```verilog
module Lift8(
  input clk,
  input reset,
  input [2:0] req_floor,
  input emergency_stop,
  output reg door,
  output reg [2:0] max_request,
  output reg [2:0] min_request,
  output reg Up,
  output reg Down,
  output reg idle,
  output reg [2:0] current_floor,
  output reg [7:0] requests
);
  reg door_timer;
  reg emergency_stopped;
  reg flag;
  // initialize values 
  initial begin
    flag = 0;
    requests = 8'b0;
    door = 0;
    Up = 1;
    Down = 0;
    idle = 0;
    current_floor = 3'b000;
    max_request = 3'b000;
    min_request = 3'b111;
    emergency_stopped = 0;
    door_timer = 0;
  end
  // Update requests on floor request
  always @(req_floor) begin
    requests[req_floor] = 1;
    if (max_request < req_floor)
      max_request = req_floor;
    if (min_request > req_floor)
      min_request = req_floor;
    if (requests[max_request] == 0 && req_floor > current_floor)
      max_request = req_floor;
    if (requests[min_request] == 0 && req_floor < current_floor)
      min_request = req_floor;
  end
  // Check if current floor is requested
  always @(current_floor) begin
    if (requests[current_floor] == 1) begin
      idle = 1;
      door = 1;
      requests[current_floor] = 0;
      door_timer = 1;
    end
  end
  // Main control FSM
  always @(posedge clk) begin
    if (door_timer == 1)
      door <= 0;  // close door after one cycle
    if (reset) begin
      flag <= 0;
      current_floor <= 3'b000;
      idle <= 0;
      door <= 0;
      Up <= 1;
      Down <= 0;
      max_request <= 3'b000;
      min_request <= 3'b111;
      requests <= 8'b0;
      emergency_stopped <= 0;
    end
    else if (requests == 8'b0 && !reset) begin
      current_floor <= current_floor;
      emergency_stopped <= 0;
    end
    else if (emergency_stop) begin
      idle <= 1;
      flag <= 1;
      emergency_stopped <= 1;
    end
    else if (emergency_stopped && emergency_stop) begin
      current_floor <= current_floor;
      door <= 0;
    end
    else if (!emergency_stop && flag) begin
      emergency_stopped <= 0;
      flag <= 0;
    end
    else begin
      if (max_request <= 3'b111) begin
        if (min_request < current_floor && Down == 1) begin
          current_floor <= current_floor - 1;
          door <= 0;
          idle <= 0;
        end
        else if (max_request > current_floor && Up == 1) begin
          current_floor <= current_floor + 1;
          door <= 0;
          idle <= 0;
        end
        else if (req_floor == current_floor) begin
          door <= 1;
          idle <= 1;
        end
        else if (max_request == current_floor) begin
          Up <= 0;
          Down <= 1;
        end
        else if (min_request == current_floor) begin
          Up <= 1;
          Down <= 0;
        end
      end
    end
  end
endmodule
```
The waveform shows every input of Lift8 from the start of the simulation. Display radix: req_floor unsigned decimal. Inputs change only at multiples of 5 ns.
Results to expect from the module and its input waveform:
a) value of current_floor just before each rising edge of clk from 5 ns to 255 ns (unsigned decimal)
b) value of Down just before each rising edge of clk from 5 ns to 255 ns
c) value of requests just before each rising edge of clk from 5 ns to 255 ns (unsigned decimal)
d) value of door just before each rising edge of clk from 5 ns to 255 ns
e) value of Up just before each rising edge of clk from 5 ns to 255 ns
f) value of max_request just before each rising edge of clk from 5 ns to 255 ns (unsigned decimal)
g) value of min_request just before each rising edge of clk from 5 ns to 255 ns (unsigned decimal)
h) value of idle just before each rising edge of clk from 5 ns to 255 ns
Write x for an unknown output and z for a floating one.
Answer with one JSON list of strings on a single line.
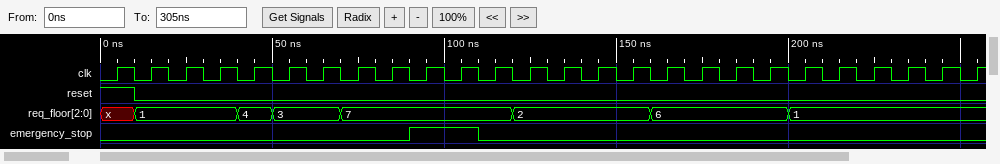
["0, 0, 1, 1, 1, 2, 3, 4, 5, 6, 6, 6, 6, 7, 7, 6, 5, 4, 3, 2, 2, 3, 4, 5, 6, 6", "0 0 0 0 0 0 0 0 0 0 0 0 0 0 1 1 1 1 1 1 0 0 0 0 0 1", "0, 2, 0, 0, 16, 24, 16, 128, 128, 128, 128, 128, 132, 4, 4, 4, 68, 68, 68, 64, 66, 66, 66, 66, 2, 2", "0 0 1 0 0 0 1 1 0 0 0 0 0 1 0 0 0 0 0 1 0 0 0 0 1 0", "1 1 1 1 1 1 1 1 1 1 1 1 1 1 0 0 0 0 0 0 1 1 1 1 1 0", "0, 1, 1, 1, 4, 4, 4, 7, 7, 7, 7, 7, 7, 7, 7, 7, 6, 6, 6, 6, 6, 6, 6, 6, 6, 6", "7, 1, 1, 1, 1, 1, 1, 1, 1, 1, 1, 1, 2, 2, 2, 2, 2, 2, 2, 2, 1, 1, 1, 1, 1, 1", "0 0 1 1 1 0 1 1 0 0 1 1 1 1 1 0 0 0 0 1 1 0 0 0 1 1"]
